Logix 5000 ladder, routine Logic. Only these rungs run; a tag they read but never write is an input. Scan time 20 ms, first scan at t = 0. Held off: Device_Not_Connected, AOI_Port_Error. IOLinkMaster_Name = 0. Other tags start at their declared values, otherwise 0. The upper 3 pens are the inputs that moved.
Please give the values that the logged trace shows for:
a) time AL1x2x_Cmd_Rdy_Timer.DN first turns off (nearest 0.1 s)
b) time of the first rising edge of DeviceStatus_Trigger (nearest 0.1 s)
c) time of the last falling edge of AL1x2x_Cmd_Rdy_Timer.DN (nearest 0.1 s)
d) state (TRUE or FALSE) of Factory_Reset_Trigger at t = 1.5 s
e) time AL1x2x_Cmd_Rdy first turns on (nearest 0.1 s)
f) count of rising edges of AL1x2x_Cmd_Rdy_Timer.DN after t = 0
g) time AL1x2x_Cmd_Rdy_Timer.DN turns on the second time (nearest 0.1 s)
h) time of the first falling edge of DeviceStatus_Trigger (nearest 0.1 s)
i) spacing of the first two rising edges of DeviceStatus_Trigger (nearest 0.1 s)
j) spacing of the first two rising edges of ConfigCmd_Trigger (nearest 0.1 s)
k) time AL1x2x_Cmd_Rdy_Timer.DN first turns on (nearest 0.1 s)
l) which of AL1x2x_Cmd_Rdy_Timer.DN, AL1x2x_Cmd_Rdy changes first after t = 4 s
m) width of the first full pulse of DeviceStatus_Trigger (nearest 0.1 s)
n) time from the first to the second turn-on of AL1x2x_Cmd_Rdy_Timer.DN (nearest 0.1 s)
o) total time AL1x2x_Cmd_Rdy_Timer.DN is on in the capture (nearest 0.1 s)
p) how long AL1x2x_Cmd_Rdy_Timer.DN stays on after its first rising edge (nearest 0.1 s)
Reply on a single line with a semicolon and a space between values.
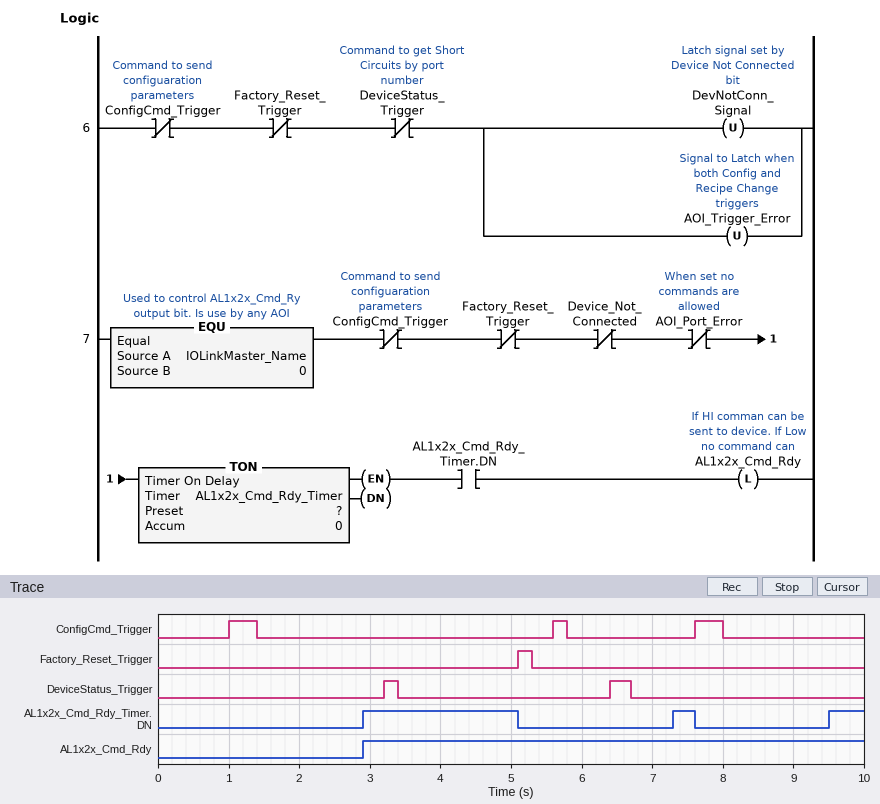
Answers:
5.1 s; 3.2 s; 7.6 s; FALSE; 2.9 s; 3; 7.3 s; 3.4 s; 3.2 s; 4.6 s; 2.9 s; AL1x2x_Cmd_Rdy_Timer.DN; 0.2 s; 4.4 s; 3.0 s; 2.2 s
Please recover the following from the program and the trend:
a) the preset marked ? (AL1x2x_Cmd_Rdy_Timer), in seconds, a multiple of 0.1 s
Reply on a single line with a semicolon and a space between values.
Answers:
1.5 s
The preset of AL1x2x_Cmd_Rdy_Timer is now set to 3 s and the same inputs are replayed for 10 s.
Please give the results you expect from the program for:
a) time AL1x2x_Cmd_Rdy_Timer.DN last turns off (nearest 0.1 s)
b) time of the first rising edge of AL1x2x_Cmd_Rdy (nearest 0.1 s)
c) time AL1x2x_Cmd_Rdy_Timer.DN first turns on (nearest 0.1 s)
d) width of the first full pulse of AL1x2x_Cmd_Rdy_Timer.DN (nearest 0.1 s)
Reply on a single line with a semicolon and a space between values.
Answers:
5.1 s; 4.4 s; 4.4 s; 0.7 s
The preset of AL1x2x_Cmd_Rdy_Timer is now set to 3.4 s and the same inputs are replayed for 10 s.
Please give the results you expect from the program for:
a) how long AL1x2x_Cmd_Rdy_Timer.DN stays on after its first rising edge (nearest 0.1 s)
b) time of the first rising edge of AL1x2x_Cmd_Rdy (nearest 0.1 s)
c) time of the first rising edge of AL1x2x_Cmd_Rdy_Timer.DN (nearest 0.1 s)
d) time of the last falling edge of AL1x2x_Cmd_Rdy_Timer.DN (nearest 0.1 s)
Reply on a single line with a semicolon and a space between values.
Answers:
0.3 s; 4.8 s; 4.8 s; 5.1 s
